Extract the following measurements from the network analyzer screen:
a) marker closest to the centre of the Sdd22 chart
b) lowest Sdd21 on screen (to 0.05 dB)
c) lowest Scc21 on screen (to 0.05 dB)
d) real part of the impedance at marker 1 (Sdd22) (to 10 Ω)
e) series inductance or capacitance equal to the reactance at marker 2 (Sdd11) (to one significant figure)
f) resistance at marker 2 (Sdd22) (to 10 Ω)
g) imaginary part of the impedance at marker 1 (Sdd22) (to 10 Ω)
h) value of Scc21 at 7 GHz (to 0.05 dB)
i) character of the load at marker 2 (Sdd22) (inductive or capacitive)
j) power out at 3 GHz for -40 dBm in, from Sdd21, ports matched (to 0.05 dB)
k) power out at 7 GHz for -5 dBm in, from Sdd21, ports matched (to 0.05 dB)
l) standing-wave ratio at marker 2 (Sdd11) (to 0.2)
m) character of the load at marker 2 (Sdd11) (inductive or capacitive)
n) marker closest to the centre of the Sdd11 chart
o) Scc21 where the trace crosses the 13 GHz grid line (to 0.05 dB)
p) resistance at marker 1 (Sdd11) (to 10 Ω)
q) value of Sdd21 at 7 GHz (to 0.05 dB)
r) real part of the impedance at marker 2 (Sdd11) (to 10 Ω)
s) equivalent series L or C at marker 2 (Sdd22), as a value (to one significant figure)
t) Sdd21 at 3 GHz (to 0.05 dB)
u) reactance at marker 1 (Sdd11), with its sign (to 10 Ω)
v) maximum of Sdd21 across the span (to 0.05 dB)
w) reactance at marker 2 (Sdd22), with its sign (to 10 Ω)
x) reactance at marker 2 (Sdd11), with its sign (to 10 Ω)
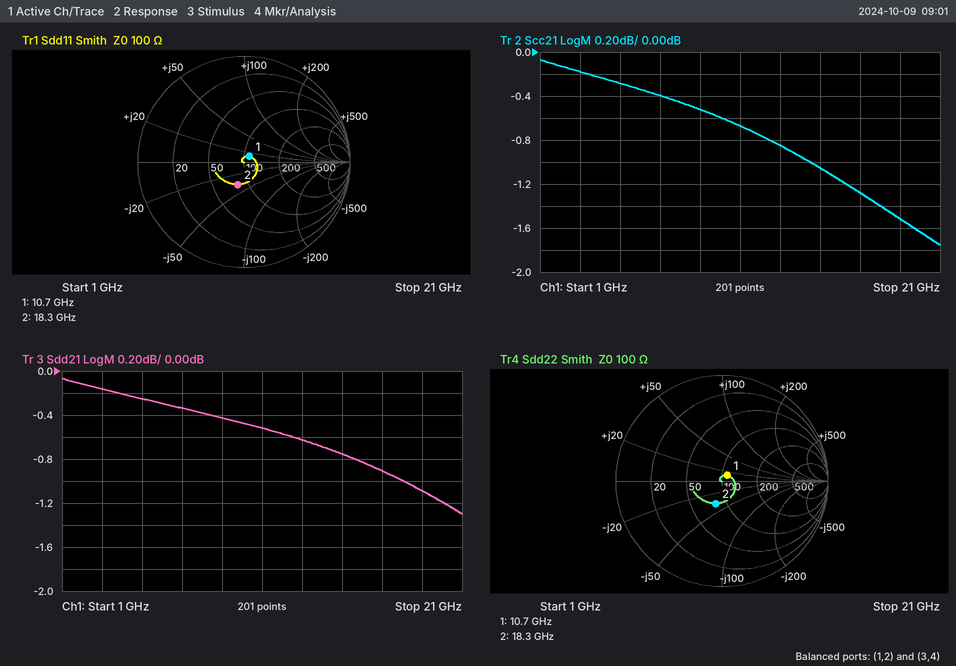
marker 1
-1.30 dB
-1.75 dB
110 Ω
200 fF
80 Ω
+10 Ω
-0.40 dB
capacitive
-40.15 dBm
-5.35 dBm
1.6
capacitive
marker 1
-0.85 dB
110 Ω
-0.35 dB
80 Ω
200 fF
-0.15 dB
+10 Ω
-0.05 dB
-40 Ω
-40 Ω
